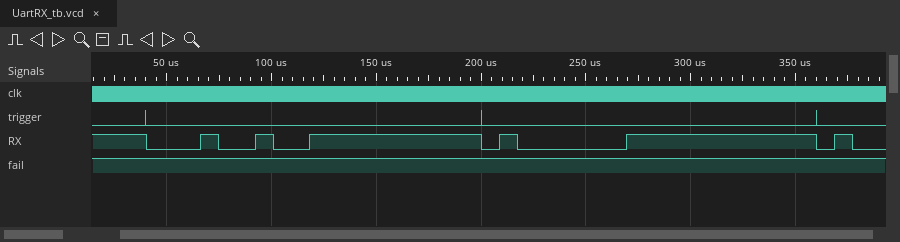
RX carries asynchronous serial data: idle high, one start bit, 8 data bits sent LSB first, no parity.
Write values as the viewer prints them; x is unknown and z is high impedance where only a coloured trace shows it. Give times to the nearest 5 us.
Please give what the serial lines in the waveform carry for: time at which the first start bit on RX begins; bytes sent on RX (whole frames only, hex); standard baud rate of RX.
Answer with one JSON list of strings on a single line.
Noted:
["40 us", "24, 81", "115200 baud"]
